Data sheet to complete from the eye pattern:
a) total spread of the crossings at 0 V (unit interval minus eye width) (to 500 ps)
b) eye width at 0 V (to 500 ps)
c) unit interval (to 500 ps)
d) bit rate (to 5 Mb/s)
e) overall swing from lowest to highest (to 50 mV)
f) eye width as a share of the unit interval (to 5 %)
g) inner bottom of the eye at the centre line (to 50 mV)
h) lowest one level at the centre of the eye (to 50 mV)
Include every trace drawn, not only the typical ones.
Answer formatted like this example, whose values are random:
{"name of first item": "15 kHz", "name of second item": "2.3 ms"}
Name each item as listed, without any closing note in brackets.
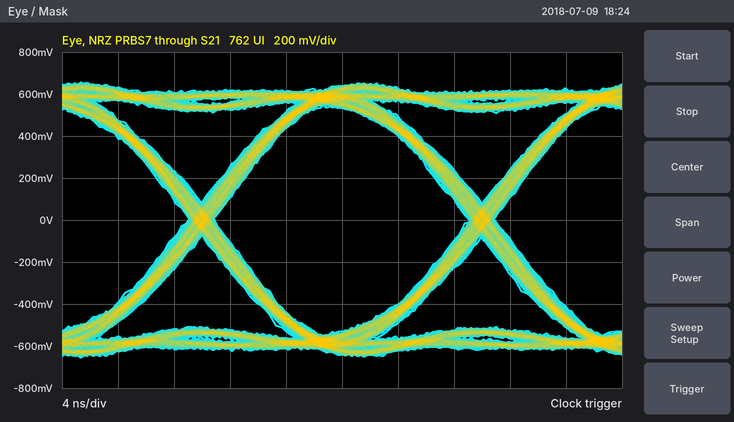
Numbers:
{"total spread of the crossings at 0 V (unit interval minus eye width)": "2.0 ns", "eye width at 0 V": "18.0 ns", "unit interval": "20.0 ns", "bit rate": "50 Mb/s", "overall swing from lowest to highest": "1.30 V", "eye width as a share of the unit interval": "90 %", "inner bottom of the eye at the centre line": "-550 mV", "lowest one level at the centre of the eye": "550 mV"}
